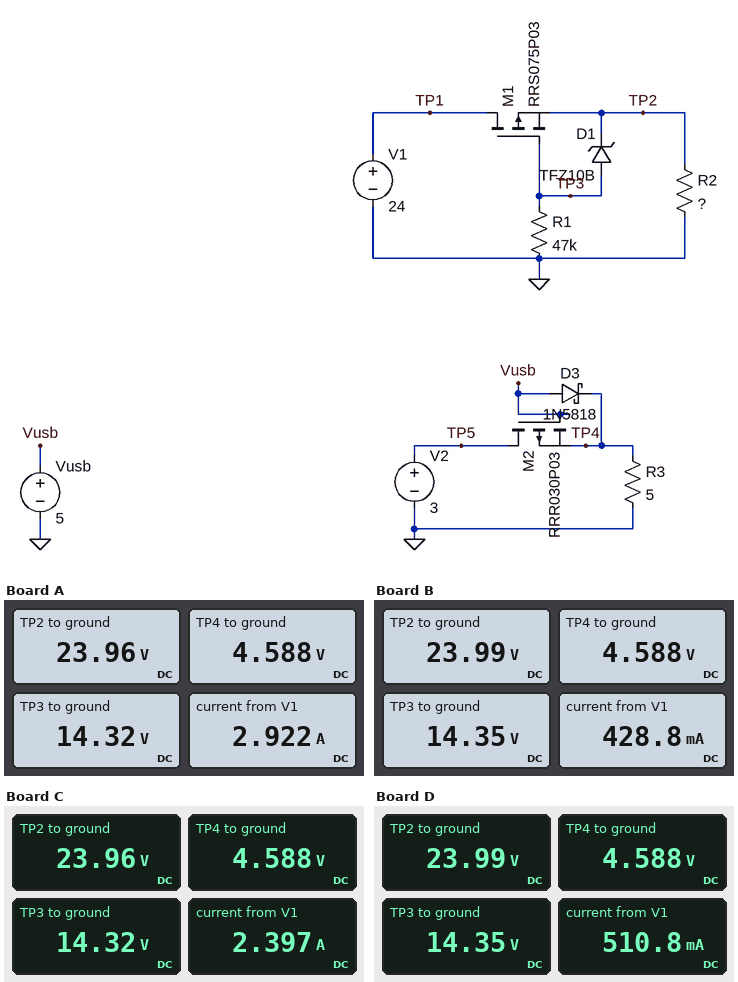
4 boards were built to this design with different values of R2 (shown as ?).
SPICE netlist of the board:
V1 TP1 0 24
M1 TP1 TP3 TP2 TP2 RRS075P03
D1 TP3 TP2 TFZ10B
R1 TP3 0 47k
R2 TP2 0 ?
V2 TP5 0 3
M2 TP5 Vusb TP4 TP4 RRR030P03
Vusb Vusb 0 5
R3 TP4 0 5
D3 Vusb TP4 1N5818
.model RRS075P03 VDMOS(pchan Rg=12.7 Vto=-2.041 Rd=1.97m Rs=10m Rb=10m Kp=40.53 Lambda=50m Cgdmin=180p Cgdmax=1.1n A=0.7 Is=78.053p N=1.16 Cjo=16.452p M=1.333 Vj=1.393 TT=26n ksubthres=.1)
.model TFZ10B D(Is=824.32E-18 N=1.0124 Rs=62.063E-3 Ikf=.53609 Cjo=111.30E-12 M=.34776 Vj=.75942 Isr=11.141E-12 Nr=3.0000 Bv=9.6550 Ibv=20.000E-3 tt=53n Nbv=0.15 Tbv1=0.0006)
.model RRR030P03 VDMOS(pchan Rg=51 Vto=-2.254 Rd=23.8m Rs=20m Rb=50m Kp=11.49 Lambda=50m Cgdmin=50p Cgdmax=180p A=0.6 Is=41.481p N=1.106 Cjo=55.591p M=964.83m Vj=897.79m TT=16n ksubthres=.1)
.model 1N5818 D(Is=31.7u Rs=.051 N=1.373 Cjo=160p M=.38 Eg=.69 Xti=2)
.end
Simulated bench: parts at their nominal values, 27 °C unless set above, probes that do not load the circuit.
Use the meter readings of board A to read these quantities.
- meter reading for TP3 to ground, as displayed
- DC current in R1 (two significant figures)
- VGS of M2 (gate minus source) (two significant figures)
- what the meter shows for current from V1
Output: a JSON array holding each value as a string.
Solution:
["14.32 V", "300 µA", "410 mV", "2.922 A"]
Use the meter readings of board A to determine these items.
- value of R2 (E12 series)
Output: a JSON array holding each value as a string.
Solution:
["8.2 Ω"]
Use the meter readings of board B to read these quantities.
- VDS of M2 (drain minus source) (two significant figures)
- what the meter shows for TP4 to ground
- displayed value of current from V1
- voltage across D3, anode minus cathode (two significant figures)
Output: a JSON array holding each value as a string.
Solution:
["-1.6 V", "4.588 V", "428.8 mA", "410 mV"]
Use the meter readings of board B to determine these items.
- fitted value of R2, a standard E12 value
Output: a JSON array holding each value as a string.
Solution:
["56 Ω"]
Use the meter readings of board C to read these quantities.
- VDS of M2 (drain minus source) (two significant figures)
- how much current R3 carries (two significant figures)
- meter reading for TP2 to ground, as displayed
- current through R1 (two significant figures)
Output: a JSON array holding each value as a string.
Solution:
["-1.6 V", "920 mA", "23.96 V", "300 µA"]
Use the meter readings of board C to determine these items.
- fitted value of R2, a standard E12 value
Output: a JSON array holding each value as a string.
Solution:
["10 Ω"]
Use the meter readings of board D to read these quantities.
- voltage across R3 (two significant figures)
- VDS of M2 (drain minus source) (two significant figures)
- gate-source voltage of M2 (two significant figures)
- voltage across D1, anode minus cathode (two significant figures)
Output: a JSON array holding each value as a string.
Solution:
["4.6 V", "-1.6 V", "410 mV", "-9.6 V"]
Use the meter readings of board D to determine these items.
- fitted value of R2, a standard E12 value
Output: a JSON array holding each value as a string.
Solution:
["47 Ω"]
